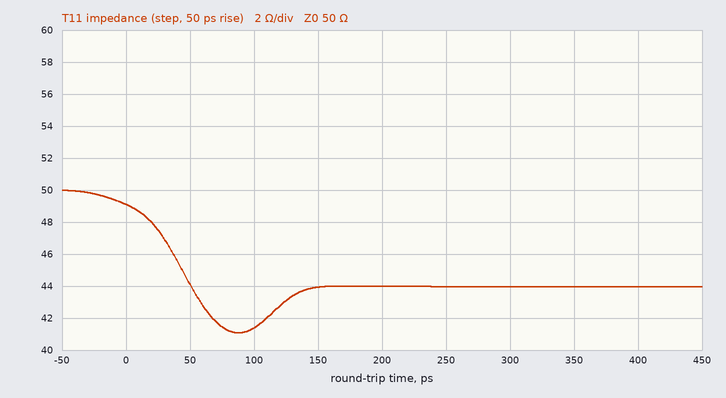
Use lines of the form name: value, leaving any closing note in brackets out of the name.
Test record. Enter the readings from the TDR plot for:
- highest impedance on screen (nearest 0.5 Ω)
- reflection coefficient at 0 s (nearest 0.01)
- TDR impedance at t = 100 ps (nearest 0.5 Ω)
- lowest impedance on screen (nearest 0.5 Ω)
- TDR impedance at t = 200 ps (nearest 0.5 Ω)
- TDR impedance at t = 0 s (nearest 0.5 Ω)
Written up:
highest impedance on screen: 50.0 Ω
reflection coefficient at 0 s: -0.01
TDR impedance at t = 100 ps: 41.5 Ω
lowest impedance on screen: 41.0 Ω
TDR impedance at t = 200 ps: 44.0 Ω
TDR impedance at t = 0 s: 49.0 Ω
